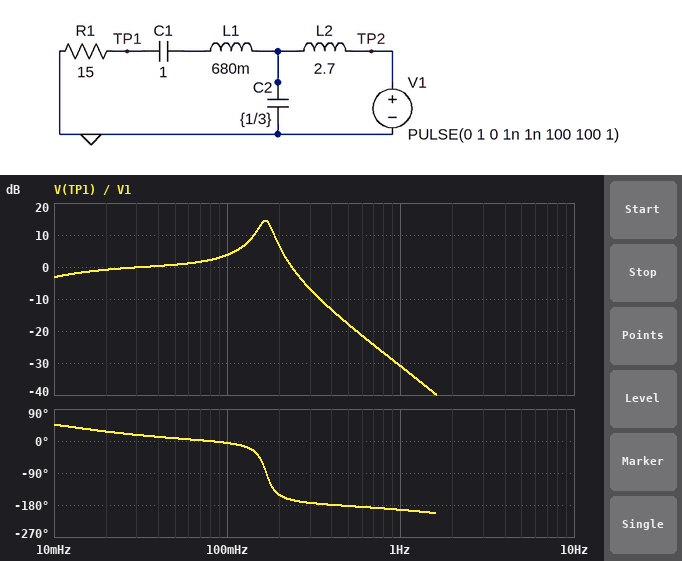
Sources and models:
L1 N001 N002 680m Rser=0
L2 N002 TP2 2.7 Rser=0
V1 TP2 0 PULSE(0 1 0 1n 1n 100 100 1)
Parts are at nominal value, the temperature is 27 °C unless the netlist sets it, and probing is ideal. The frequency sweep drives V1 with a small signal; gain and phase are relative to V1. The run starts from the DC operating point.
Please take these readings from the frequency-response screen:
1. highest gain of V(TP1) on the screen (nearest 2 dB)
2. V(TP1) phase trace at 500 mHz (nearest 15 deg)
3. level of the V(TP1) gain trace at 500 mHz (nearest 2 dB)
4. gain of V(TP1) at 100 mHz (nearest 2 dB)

14 dB
-180 deg
-18 dB
4 dB
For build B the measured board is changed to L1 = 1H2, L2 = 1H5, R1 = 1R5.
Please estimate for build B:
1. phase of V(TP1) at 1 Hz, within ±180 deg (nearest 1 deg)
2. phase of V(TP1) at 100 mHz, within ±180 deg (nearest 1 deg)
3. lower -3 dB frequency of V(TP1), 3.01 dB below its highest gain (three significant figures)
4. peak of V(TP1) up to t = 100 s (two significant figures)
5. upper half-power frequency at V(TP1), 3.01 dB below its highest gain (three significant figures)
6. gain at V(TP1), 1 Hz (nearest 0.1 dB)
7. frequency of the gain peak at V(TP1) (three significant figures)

102 deg
-13 deg
66.8 mHz
710 mV
157 mHz
-38.9 dB
98.4 mHz
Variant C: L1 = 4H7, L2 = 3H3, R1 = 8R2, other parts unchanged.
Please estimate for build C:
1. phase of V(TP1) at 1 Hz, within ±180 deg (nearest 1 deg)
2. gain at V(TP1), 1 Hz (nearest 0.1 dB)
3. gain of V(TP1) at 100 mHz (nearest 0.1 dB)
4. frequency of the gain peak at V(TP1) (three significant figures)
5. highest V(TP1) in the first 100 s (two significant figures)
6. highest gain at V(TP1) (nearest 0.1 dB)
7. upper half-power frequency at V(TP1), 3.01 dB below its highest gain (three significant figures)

106 deg
-43.8 dB
3.6 dB
160 mHz
1.3 V
8.6 dB
185 mHz
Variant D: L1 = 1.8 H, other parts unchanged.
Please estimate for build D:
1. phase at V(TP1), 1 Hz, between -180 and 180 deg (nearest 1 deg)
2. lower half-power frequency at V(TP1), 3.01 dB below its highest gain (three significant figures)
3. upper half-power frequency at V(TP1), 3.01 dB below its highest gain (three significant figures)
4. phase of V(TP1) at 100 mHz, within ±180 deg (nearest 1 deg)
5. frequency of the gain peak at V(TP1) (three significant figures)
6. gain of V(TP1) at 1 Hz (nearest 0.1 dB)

145 deg
150 mHz
183 mHz
-8 deg
167 mHz
-32.5 dB
